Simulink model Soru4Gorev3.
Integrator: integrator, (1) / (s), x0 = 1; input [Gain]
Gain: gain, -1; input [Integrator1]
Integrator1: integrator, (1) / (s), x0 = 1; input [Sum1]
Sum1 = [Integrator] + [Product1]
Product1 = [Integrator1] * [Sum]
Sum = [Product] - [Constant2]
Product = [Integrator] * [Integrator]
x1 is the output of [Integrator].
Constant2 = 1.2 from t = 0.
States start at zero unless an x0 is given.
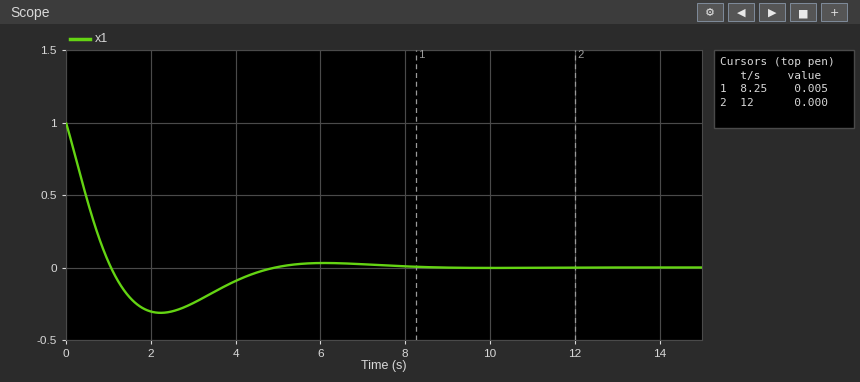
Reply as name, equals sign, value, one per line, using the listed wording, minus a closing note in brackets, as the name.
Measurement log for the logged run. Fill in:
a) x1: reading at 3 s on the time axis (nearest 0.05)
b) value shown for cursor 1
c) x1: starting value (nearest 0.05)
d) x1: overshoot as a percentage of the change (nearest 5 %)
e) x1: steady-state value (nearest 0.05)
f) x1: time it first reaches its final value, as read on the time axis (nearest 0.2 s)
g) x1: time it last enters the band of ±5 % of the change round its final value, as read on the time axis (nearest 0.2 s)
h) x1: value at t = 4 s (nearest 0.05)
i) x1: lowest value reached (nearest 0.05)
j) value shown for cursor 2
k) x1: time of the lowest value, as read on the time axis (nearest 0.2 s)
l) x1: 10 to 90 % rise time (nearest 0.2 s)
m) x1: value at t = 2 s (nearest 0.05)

x1: reading at 3 s on the time axis = -0.25
value shown for cursor 1 = 0.005
x1: starting value = 1.00
x1: overshoot as a percentage of the change = 30 %
x1: steady-state value = 0.00
x1: time it first reaches its final value, as read on the time axis = 1.0 s
x1: time it last enters the band of ±5 % of the change round its final value, as read on the time axis = 4.4 s
x1: value at t = 4 s = -0.10
x1: lowest value reached = -0.30
value shown for cursor 2 = 0.000
x1: time of the lowest value, as read on the time axis = 2.2 s
x1: 10 to 90 % rise time = 0.8 s
x1: value at t = 2 s = -0.30
